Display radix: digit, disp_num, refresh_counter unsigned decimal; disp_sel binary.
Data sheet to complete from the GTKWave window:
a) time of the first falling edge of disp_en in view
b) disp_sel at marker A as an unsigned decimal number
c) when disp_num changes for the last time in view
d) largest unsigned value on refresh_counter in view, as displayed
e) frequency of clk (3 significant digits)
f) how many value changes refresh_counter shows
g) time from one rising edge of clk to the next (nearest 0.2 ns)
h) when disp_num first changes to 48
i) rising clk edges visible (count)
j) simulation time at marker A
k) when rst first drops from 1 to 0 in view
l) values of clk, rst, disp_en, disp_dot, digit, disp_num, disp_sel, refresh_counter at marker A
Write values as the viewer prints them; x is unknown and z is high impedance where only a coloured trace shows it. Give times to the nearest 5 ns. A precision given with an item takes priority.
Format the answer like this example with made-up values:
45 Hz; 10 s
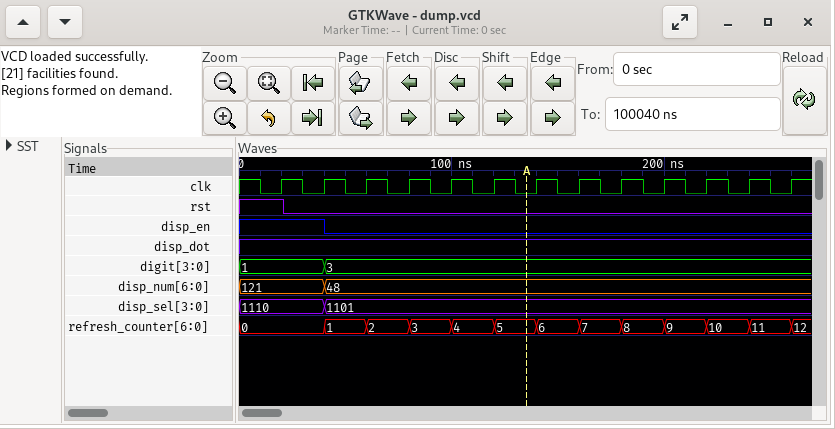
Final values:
40 ns; 13; 40 ns; 12; 50.0 MHz; 12; 20 ns; 40 ns; 13; 135 ns; 20 ns; clk=0, rst=0, disp_en=0, disp_dot=1, digit=3, disp_num=48, disp_sel=1101, refresh_counter=5
